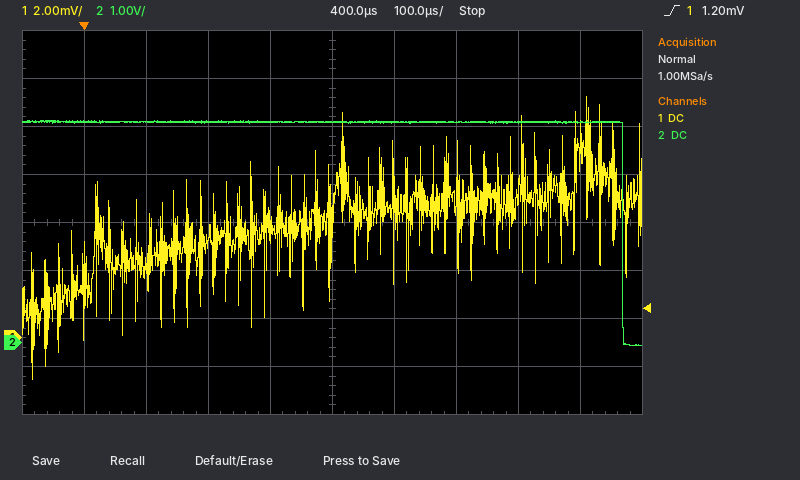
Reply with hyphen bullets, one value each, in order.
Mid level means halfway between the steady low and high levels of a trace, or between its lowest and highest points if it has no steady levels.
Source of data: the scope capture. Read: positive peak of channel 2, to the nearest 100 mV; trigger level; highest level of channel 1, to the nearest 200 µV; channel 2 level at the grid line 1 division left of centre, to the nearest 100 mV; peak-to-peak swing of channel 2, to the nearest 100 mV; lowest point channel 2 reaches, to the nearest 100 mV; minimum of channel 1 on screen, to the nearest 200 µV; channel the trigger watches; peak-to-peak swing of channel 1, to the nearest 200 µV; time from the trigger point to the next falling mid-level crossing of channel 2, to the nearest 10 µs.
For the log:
- 4.6 V
- 1.20 mV
- 10.0 mV
- 4.6 V
- 4.7 V
- -100 mV
- -1.8 mV
- channel 1
- 11.8 mV
- 870 µs
